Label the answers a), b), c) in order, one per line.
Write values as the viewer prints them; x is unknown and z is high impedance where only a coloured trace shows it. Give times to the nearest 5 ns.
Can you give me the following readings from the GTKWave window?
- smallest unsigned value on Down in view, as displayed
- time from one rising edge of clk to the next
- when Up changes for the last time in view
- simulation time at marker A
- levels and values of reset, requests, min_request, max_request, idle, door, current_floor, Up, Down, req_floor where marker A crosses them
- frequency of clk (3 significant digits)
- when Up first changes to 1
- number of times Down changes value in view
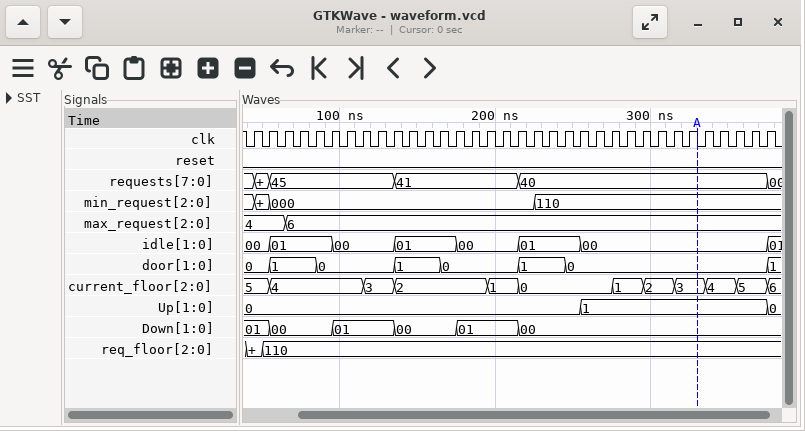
a) 00
b) 10 ns
c) 375 ns
d) 330 ns
e) reset=0, requests=40, min_request=110, max_request=6, idle=00, door=0, current_floor=3, Up=1, Down=00, req_floor=110
f) 100 MHz
g) 255 ns
h) 5
